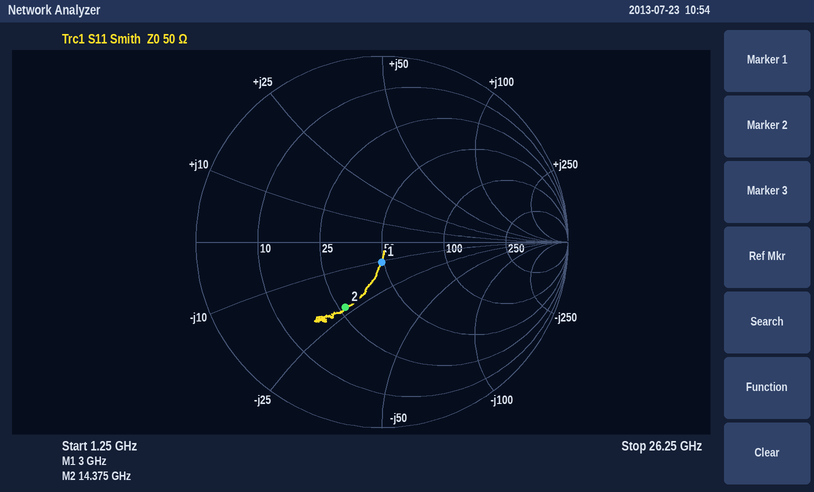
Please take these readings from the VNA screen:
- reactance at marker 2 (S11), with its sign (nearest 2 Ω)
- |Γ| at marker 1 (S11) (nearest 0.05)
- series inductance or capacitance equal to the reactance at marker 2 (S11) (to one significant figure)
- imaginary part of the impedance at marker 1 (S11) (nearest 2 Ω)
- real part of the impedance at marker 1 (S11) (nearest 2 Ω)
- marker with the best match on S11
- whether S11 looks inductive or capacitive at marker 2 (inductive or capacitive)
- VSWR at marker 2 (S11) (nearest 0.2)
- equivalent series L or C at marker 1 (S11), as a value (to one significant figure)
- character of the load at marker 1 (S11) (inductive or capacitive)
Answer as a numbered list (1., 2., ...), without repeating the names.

1. -22 Ω
2. 0.10
3. 500 fF
4. -10 Ω
5. 48 Ω
6. marker 1
7. capacitive
8. 2.4
9. 5 pF
10. capacitive
